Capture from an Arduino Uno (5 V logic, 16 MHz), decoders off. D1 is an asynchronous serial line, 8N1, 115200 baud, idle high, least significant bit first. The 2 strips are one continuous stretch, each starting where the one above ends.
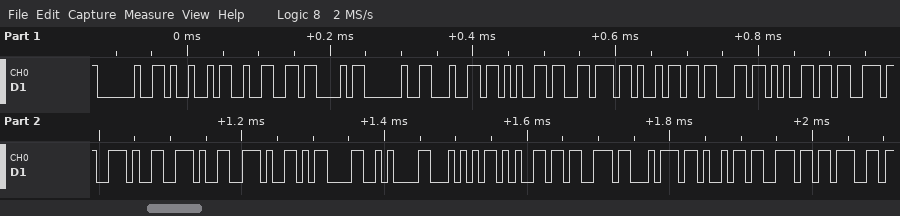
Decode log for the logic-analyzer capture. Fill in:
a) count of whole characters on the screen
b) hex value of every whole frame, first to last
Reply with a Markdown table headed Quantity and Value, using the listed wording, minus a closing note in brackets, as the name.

| Quantity | Value |
|---|---|
| count of whole characters on the screen | 24 |
| hex value of every whole frame, first to last | 20 49 32 43 20 64 65 76 69 63 65 73 2E 2E 2E 0D 0A 54 65 73 74 69 6E 67 |
